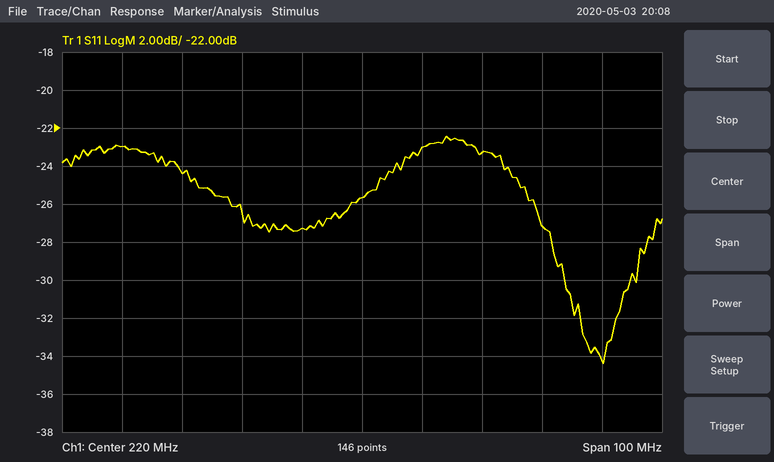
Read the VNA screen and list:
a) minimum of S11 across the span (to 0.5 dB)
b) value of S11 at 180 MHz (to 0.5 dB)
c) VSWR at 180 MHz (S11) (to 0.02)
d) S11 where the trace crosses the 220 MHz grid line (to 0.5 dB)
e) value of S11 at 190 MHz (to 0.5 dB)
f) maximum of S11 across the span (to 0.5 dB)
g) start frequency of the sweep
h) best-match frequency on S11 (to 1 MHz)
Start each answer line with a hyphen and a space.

- -34.5 dB
- -23.0 dB
- 1.16
- -25.5 dB
- -24.5 dB
- -22.5 dB
- 170 MHz
- 260 MHz
